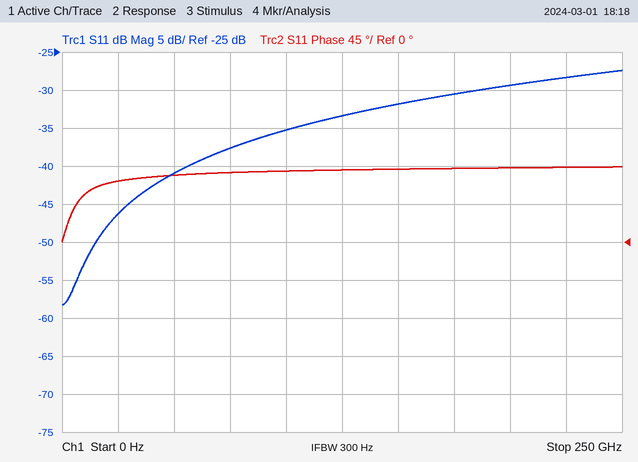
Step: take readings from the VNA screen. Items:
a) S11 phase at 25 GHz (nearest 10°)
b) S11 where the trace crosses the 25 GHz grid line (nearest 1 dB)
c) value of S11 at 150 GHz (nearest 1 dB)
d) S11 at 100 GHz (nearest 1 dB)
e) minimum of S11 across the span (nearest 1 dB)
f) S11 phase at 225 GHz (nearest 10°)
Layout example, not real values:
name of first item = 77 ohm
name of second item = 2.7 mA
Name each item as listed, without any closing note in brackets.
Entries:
S11 phase at 25 GHz = 70°
S11 where the trace crosses the 25 GHz grid line = -46 dB
value of S11 at 150 GHz = -32 dB
S11 at 100 GHz = -35 dB
minimum of S11 across the span = -58 dB
S11 phase at 225 GHz = 90°
